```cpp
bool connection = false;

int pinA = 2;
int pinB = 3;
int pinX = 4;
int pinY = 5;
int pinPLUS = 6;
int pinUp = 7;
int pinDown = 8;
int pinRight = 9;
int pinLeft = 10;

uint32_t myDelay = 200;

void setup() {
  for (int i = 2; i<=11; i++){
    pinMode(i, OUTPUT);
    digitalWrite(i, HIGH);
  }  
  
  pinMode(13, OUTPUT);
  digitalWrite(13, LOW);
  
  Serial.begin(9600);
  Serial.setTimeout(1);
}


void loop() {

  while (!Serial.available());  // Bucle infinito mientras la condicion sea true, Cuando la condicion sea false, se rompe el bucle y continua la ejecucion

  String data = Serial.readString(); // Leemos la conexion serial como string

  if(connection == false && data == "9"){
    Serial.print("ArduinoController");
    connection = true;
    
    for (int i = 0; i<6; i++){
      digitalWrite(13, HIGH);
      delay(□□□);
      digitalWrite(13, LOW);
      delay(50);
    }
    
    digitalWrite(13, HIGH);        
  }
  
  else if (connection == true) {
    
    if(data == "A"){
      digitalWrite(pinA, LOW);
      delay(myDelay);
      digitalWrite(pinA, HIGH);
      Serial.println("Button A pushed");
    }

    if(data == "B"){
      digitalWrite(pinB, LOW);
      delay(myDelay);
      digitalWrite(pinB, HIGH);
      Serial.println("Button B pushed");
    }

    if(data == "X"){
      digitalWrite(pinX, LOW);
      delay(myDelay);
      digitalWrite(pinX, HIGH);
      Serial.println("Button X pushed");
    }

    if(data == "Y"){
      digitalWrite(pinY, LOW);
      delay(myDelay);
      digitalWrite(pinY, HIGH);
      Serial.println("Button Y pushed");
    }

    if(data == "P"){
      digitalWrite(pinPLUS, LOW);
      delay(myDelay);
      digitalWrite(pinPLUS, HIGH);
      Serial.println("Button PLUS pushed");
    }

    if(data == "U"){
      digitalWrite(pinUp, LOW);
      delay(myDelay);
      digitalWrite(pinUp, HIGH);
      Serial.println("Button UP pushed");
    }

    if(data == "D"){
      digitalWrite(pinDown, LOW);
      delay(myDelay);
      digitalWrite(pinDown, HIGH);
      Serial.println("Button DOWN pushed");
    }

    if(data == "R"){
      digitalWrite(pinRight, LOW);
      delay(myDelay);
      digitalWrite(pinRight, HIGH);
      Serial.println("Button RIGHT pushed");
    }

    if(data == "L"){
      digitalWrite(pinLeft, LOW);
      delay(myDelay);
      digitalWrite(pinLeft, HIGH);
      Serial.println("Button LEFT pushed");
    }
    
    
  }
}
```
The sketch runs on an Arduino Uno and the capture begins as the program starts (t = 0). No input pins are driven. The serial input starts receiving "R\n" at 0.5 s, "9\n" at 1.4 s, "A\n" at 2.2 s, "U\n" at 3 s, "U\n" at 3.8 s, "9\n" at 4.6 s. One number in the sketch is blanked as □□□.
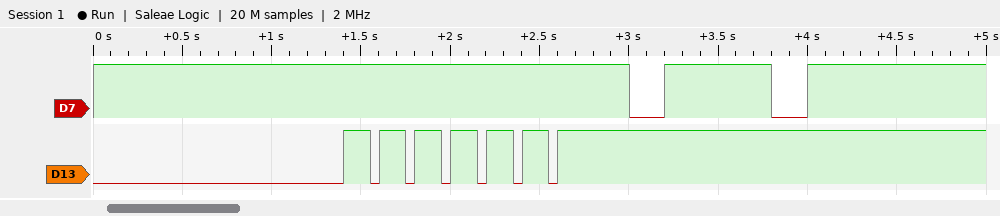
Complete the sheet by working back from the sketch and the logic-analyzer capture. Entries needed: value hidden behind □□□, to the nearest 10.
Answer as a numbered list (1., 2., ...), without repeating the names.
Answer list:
1. 150
